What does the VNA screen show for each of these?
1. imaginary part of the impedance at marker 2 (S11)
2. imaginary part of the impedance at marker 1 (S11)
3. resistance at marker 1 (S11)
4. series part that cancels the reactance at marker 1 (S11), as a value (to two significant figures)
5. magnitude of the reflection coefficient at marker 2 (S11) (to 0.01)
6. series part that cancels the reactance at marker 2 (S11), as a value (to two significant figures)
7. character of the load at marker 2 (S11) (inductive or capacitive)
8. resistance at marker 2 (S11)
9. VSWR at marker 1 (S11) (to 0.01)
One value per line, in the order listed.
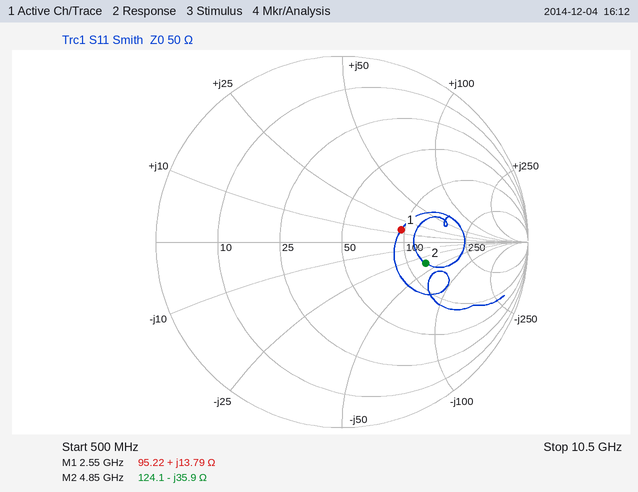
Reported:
-35.9 Ω
+13.79 Ω
95.22 Ω
4.5 pF
0.46
1.2 nH
capacitive
124.1 Ω
1.96
